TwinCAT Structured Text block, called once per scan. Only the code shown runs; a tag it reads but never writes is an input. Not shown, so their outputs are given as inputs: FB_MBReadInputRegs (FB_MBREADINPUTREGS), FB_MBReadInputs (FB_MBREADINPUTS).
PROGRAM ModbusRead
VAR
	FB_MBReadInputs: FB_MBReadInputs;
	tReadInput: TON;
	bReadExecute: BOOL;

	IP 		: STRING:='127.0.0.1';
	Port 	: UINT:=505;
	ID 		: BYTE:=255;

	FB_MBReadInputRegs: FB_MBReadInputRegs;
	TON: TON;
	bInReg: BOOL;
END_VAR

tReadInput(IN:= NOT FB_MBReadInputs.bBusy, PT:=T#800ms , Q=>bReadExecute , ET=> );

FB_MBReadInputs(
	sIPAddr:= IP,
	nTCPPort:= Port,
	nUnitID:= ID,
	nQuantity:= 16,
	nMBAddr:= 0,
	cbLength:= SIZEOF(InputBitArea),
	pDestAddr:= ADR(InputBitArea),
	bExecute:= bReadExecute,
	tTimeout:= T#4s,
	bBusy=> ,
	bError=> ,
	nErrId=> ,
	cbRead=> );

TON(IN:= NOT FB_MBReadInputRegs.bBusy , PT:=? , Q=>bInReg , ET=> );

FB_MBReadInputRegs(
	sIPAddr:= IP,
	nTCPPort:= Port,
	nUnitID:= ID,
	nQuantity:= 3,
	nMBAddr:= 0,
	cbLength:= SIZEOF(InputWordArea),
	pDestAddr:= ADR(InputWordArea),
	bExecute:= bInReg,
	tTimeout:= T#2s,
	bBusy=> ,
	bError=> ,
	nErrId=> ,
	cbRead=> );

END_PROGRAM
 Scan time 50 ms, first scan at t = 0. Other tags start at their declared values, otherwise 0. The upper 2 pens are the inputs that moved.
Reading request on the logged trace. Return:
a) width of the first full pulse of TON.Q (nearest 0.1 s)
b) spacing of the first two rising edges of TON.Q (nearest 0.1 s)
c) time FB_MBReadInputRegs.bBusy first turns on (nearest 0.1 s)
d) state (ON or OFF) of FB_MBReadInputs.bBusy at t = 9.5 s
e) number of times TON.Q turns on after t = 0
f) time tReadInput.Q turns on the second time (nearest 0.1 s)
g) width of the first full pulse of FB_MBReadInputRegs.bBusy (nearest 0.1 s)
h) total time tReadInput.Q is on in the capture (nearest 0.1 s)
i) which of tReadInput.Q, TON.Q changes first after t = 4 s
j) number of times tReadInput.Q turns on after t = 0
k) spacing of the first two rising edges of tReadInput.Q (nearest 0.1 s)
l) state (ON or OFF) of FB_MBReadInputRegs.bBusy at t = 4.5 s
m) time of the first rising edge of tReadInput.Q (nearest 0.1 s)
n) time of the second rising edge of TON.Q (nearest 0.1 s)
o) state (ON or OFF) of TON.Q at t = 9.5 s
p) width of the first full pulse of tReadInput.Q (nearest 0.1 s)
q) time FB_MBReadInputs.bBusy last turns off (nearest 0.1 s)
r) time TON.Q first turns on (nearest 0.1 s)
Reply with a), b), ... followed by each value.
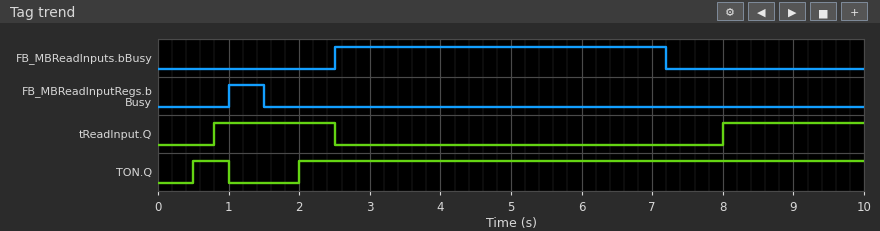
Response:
a) 0.5 s
b) 1.5 s
c) 1.0 s
d) OFF
e) 2
f) 8.0 s
g) 0.5 s
h) 3.7 s
i) tReadInput.Q
j) 2
k) 7.2 s
l) OFF
m) 0.8 s
n) 2.0 s
o) ON
p) 1.7 s
q) 7.2 s
r) 0.5 s
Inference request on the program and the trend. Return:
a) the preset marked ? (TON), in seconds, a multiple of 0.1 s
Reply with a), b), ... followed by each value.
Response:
a) 0.5 s
